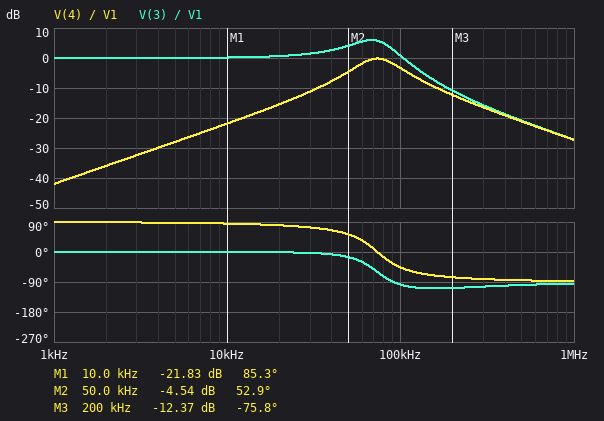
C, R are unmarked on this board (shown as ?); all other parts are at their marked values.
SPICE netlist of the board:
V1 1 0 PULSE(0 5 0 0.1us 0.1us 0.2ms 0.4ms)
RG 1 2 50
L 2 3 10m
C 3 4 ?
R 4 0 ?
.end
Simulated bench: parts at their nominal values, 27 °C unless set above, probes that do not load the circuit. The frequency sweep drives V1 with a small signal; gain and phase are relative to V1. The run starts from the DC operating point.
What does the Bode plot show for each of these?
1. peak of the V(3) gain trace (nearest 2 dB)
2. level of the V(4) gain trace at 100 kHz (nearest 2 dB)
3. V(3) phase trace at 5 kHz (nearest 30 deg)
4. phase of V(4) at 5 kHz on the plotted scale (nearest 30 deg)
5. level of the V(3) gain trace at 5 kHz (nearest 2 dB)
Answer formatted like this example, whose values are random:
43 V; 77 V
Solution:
6 dB; -4 dB; 0 deg; 90 deg; 0 dB
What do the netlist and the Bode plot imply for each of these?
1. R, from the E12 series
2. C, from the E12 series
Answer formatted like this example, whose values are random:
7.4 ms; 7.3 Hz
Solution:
2.7 kΩ; 470 pF
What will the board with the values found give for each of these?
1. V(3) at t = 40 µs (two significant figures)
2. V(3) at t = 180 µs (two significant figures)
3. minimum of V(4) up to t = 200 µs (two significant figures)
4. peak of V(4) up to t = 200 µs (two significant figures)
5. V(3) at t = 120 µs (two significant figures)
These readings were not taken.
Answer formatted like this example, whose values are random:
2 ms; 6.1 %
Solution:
5.0 V; 5.0 V; -740 mV; 2.0 V; 5.0 V
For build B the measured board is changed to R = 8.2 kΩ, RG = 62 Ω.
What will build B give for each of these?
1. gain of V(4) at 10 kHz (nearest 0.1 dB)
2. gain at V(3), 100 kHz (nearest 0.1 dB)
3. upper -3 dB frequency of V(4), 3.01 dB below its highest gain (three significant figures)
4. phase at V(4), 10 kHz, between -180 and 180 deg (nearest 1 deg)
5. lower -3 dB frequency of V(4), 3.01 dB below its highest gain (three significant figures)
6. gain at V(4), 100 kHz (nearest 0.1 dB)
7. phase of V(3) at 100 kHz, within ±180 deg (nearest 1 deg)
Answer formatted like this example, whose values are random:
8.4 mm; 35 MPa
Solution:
-12.4 dB; 0.1 dB; 164 kHz; 76 deg; 32.8 kHz; -0.6 dB; -42 deg
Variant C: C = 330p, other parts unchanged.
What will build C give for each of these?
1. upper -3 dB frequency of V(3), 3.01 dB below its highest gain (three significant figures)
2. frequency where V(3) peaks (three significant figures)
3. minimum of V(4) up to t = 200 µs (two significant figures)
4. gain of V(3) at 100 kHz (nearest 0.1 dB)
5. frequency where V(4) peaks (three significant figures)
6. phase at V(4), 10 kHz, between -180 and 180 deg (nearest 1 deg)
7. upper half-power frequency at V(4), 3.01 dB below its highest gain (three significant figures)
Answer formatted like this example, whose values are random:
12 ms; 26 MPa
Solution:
104 kHz; 83.0 kHz; -780 mV; 5.0 dB; 87.6 kHz; 87 deg; 112 kHz
